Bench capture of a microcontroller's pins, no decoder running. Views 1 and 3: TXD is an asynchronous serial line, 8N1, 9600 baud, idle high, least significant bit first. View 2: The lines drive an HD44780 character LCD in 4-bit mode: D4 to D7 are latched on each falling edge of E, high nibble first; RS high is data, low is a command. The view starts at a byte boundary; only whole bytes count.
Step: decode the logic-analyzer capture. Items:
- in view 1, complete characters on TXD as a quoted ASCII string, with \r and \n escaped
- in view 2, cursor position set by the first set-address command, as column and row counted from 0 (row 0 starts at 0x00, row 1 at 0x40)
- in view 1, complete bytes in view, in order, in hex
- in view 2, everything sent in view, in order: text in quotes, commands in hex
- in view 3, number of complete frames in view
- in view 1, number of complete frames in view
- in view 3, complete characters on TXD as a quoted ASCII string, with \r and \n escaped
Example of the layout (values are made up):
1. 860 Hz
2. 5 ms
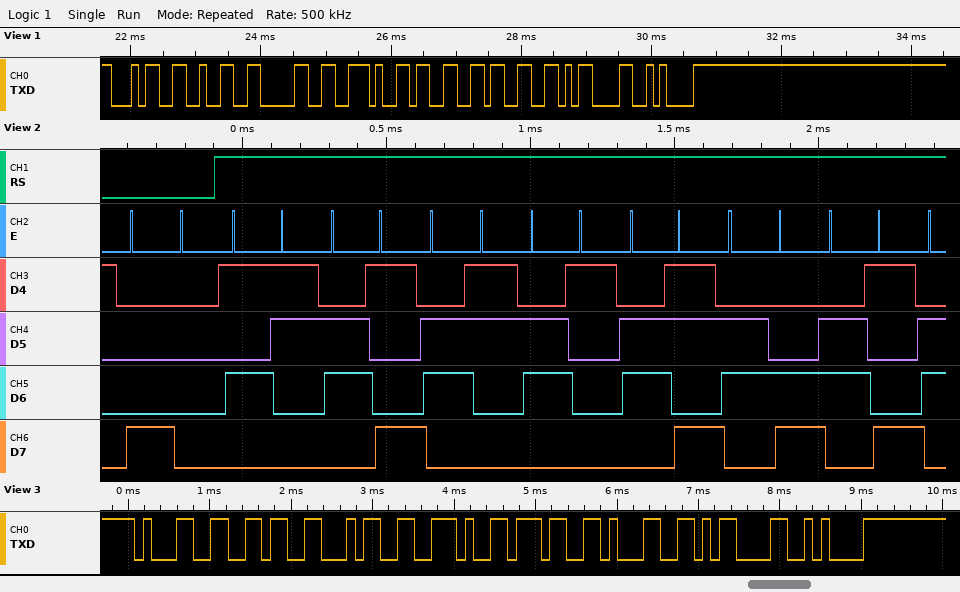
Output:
1. "420.33\r\n"
2. column 0, row 0
3. 34 32 30 2E 33 33 0D 0A
4. 0x80 "Sicakli"
5. 8
6. 8
7. "164.71\r\n"
